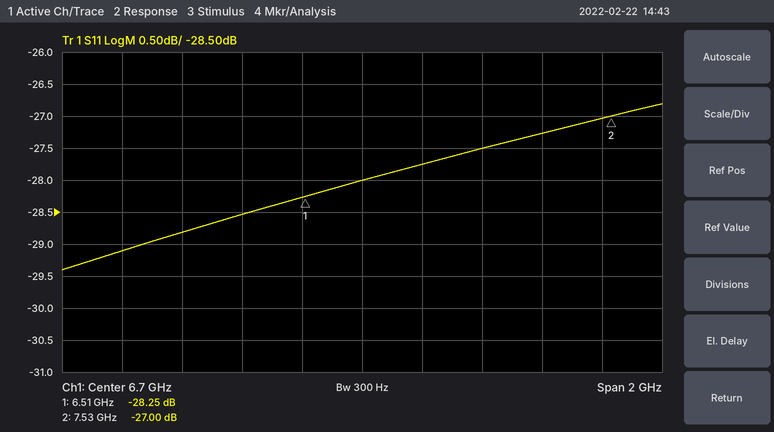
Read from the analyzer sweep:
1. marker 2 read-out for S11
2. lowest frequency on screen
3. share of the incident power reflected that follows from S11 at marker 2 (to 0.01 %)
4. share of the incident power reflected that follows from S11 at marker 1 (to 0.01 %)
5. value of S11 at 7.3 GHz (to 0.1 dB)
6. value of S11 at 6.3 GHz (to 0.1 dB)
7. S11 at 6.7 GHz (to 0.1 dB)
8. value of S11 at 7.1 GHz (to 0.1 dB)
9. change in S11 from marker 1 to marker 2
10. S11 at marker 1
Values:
-27.00 dB
5.7 GHz
0.20 %
0.15 %
-27.3 dB
-28.5 dB
-28.0 dB
-27.5 dB
1.25 dB
-28.25 dB
